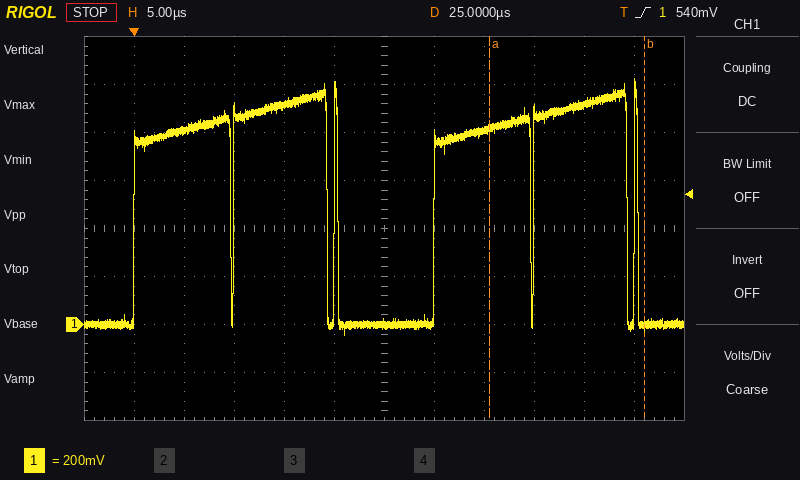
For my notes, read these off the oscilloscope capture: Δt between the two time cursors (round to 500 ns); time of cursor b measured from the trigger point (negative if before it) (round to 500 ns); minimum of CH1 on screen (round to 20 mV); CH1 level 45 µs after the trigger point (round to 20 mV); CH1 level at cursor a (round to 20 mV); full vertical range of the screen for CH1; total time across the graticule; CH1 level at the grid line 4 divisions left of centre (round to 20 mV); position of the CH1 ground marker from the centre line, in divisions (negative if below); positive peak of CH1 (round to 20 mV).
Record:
15.5 µs
+51.0 µs
-40 mV
920 mV
820 mV
1.6 V
60 µs
800 mV
-2.0 div
1.02 V
